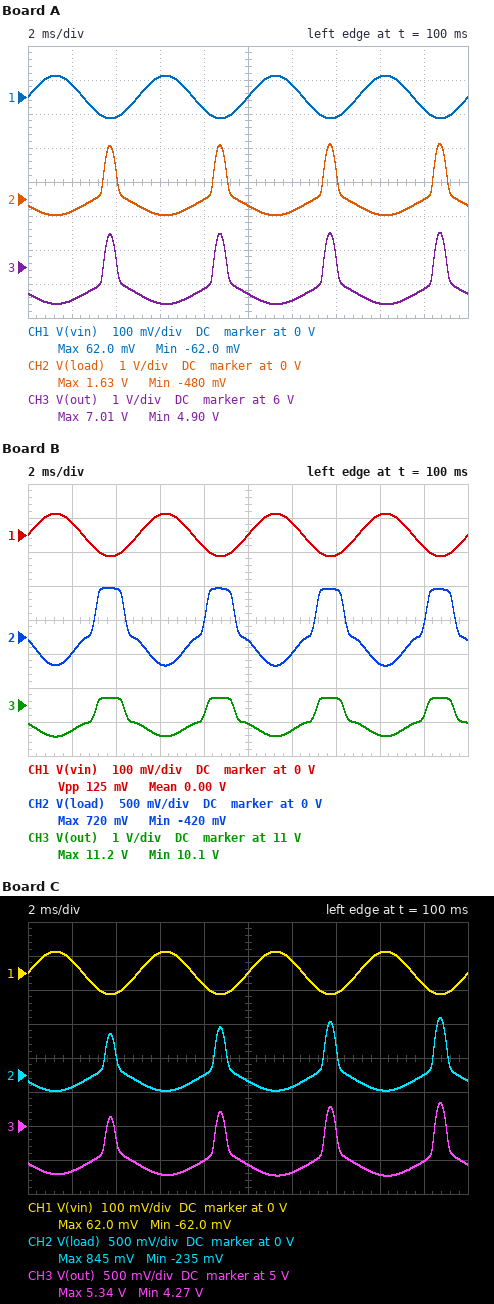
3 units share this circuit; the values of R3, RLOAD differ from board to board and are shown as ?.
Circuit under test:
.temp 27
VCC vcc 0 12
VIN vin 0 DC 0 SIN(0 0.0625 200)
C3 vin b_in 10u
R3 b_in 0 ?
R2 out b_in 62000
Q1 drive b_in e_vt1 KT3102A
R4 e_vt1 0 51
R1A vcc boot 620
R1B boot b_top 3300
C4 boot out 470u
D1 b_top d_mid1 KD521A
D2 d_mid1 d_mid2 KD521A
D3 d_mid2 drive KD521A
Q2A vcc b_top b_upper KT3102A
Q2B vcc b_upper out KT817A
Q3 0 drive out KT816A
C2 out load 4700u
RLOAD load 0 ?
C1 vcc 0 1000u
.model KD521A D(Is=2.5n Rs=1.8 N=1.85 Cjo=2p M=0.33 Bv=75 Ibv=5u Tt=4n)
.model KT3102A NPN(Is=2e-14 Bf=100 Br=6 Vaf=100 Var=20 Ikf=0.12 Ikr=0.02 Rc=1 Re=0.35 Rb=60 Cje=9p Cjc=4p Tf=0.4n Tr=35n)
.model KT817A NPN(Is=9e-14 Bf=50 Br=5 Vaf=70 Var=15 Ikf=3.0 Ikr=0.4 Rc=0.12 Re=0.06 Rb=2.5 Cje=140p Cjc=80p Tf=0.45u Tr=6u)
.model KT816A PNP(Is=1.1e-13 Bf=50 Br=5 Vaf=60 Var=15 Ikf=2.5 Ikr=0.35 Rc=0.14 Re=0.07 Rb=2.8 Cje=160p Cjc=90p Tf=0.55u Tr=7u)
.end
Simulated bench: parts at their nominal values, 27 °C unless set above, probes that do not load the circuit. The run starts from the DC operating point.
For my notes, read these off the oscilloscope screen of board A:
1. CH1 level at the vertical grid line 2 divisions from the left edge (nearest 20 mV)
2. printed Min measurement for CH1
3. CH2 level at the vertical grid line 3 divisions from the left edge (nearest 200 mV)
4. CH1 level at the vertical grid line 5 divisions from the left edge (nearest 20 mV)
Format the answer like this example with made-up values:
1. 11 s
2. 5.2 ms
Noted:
1. -60 mV
2. -62.0 mV
3. -400 mV
4. 0 V
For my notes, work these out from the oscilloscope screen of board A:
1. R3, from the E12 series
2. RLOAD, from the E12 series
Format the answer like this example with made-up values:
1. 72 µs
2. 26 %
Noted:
1. 15 kΩ
2. 5.6 Ω
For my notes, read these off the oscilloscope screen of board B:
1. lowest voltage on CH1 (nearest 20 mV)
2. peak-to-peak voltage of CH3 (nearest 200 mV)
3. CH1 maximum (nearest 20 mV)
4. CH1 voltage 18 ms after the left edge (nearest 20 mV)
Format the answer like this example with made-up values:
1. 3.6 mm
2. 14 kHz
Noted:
1. -60 mV
2. 1.2 V
3. 60 mV
4. -40 mV
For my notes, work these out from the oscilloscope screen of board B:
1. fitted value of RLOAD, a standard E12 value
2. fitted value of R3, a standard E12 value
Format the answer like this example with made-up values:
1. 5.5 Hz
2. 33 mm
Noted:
1. 12 Ω
2. 3.9 kΩ
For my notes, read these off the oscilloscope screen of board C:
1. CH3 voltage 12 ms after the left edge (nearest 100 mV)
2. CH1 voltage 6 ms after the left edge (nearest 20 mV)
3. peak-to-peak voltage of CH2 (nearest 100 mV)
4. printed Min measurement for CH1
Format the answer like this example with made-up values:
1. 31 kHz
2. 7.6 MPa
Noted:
1. 4.3 V
2. 60 mV
3. 1.1 V
4. -62.0 mV
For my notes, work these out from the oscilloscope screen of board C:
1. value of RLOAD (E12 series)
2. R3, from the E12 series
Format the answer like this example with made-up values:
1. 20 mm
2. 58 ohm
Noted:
1. 2.7 Ω
2. 22 kΩ
